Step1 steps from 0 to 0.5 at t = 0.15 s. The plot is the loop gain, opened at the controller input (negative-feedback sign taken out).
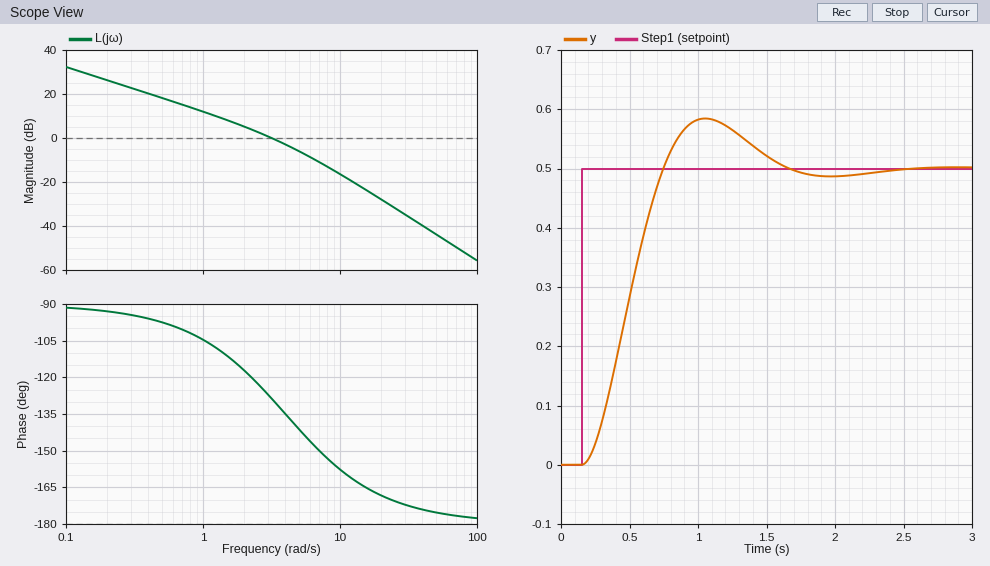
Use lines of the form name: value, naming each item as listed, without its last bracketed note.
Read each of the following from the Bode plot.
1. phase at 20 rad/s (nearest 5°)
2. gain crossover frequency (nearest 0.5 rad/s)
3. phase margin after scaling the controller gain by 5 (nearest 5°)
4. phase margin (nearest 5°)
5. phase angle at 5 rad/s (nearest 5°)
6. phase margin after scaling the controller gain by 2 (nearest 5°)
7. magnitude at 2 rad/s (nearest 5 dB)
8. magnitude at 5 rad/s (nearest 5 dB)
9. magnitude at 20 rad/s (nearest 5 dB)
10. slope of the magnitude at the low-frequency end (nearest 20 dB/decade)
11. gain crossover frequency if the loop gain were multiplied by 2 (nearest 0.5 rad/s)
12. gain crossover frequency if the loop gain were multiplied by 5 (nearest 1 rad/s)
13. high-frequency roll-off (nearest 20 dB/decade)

phase at 20 rad/s: -170°
gain crossover frequency: 3.0 rad/s
phase margin after scaling the controller gain by 5: 25°
phase margin: 50°
phase angle at 5 rad/s: -140°
phase margin after scaling the controller gain by 2: 40°
magnitude at 2 rad/s: 5 dB
magnitude at 5 rad/s: -5 dB
magnitude at 20 rad/s: -30 dB
slope of the magnitude at the low-frequency end: -20 dB/decade
gain crossover frequency if the loop gain were multiplied by 2: 5.0 rad/s
gain crossover frequency if the loop gain were multiplied by 5: 9 rad/s
high-frequency roll-off: -40 dB/decade
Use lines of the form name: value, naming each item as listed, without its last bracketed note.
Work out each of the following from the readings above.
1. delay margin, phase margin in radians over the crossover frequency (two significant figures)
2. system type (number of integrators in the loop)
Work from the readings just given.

delay margin, phase margin in radians over the crossover frequency: 0.29 s
system type: 1
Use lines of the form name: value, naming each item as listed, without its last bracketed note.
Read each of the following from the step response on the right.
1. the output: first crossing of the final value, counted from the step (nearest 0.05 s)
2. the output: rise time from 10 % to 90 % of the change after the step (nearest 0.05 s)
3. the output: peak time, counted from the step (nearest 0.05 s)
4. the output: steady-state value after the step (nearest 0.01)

the output: first crossing of the final value, counted from the step: 0.60 s
the output: rise time from 10 % to 90 % of the change after the step: 0.40 s
the output: peak time, counted from the step: 0.90 s
the output: steady-state value after the step: 0.50
